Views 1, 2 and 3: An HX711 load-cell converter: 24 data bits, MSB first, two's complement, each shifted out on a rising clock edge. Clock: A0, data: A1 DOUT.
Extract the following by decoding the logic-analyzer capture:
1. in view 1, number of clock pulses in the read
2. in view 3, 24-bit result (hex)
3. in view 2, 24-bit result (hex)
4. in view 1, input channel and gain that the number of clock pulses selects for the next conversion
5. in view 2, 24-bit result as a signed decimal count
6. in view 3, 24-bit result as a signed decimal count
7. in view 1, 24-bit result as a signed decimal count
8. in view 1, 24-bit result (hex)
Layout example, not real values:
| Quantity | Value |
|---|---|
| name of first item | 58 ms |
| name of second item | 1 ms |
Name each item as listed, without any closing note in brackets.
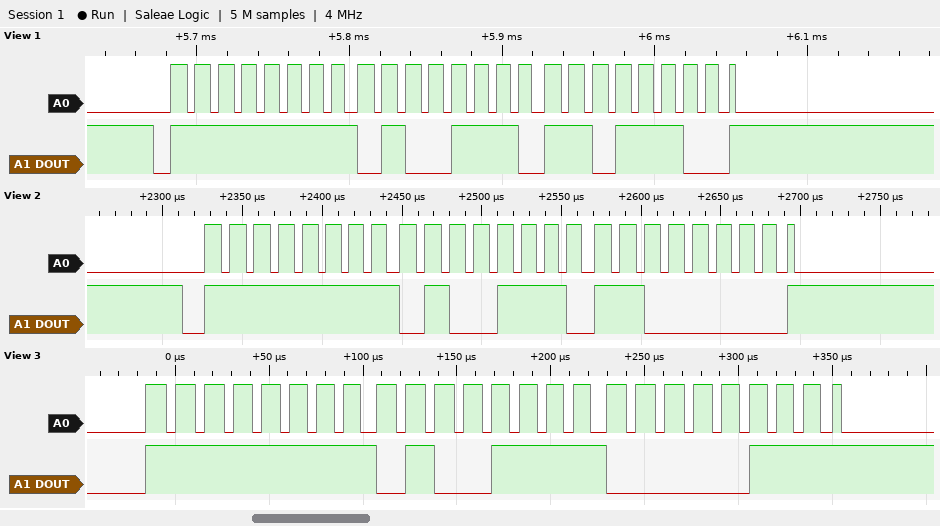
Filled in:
| Quantity | Value |
|---|---|
| in view 1, number of clock pulses in the read | 25 |
| in view 3, 24-bit result | 0xFF4F07 |
| in view 2, 24-bit result | 0xFF4EC0 |
| in view 1, input channel and gain that the number of clock pulses selects for the next conversion | channel A, gain 128 |
| in view 2, 24-bit result as a signed decimal count | -45376 |
| in view 3, 24-bit result as a signed decimal count | -45305 |
| in view 1, 24-bit result as a signed decimal count | -45348 |
| in view 1, 24-bit result | 0xFF4EDC |
